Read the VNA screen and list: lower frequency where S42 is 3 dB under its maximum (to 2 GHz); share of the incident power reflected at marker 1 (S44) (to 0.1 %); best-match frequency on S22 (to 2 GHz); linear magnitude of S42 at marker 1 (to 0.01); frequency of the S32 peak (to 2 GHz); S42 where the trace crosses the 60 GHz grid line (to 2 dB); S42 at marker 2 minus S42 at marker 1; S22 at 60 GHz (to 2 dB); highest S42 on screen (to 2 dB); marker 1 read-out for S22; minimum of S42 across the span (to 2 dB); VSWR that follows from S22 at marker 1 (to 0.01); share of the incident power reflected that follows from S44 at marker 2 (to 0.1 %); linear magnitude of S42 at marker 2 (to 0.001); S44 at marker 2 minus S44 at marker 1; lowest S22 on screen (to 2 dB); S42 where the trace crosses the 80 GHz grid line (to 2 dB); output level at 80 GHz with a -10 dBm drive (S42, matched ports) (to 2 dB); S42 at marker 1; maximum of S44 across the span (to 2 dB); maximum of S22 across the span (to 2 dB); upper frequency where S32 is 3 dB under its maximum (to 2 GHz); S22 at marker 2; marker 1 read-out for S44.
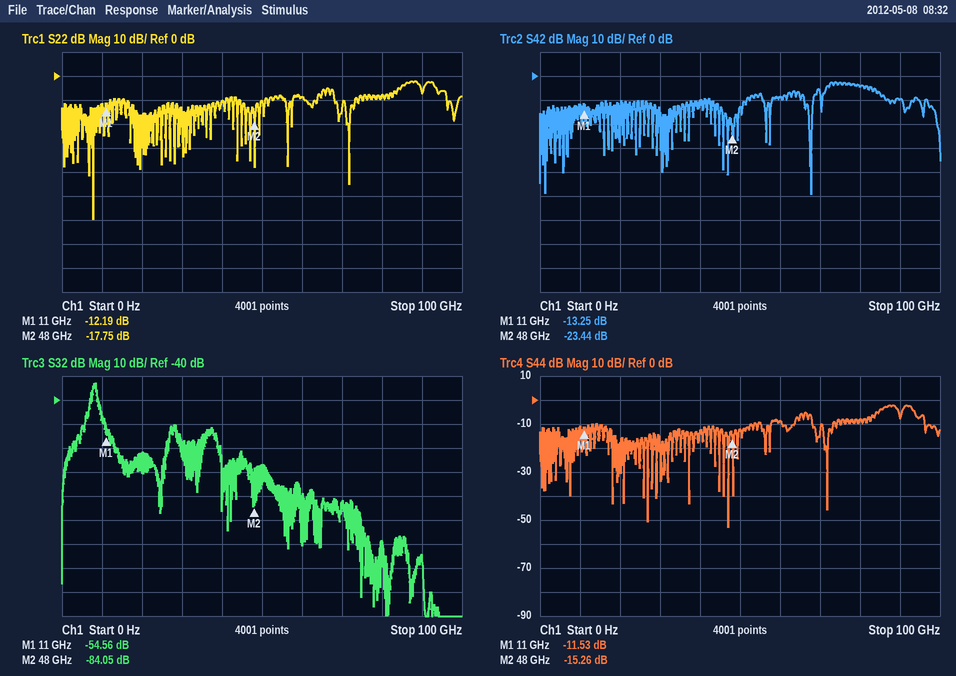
72 GHz
7.0 %
8 GHz
0.22
8 GHz
-8 dB
-10.19 dB
-8 dB
-2 dB
-12.19 dB
-50 dB
1.65
3.0 %
0.067
-3.73 dB
-60 dB
-4 dB
-14 dBm
-13.25 dB
-2 dB
-2 dB
8 GHz
-17.75 dB
-11.53 dB
